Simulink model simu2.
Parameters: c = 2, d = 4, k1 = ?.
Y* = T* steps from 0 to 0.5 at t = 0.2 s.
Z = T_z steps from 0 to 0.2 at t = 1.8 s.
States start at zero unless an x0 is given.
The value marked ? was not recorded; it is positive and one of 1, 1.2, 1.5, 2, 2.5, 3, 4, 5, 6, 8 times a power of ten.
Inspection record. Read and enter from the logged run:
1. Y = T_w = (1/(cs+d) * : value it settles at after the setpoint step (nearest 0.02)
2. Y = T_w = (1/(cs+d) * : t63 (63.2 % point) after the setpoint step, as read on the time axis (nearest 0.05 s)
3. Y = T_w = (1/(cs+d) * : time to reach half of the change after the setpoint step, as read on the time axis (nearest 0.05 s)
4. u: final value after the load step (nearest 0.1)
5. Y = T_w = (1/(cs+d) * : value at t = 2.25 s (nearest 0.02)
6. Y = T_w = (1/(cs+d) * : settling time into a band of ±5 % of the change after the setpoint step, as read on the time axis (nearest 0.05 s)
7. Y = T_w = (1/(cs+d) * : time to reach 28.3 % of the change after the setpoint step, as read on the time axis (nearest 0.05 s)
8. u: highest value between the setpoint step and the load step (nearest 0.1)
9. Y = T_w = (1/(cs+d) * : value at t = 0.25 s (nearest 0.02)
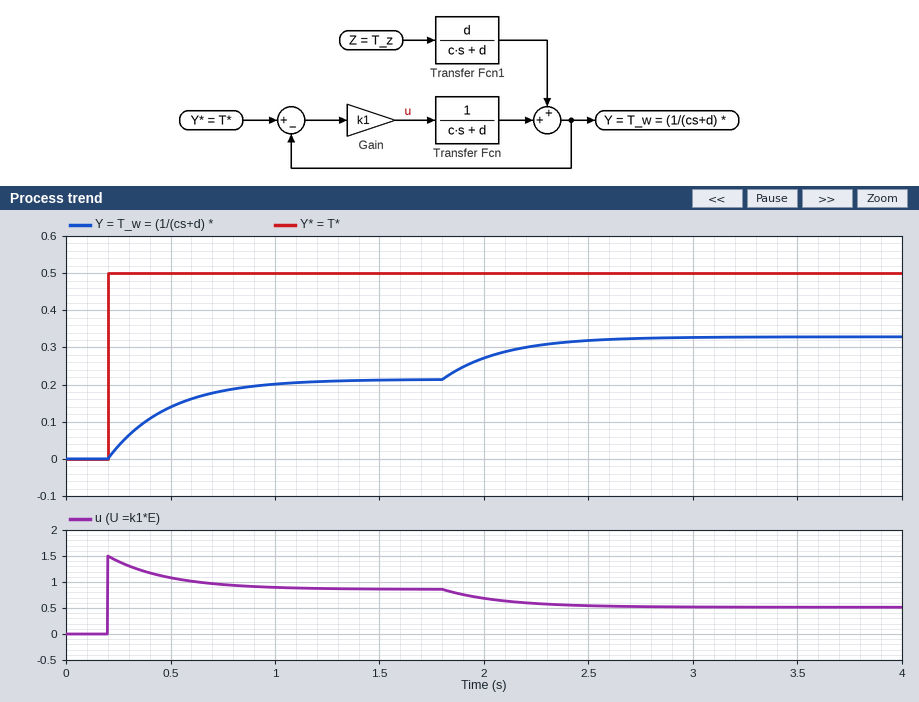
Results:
0.22
0.50 s
0.40 s
0.5
0.30
1.05 s
0.30 s
1.5
0.04
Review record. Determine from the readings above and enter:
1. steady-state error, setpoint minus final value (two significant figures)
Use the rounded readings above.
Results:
0.28
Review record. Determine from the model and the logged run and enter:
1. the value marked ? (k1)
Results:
3
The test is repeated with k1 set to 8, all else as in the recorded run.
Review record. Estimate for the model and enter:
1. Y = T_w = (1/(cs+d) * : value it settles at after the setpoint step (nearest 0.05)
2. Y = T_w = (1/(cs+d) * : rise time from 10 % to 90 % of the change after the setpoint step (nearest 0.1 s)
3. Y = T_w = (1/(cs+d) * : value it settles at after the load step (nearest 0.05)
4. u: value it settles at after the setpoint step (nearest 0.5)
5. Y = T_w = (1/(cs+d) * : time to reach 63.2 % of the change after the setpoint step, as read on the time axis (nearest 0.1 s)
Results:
0.35
0.4 s
0.40
1.5
0.4 s
